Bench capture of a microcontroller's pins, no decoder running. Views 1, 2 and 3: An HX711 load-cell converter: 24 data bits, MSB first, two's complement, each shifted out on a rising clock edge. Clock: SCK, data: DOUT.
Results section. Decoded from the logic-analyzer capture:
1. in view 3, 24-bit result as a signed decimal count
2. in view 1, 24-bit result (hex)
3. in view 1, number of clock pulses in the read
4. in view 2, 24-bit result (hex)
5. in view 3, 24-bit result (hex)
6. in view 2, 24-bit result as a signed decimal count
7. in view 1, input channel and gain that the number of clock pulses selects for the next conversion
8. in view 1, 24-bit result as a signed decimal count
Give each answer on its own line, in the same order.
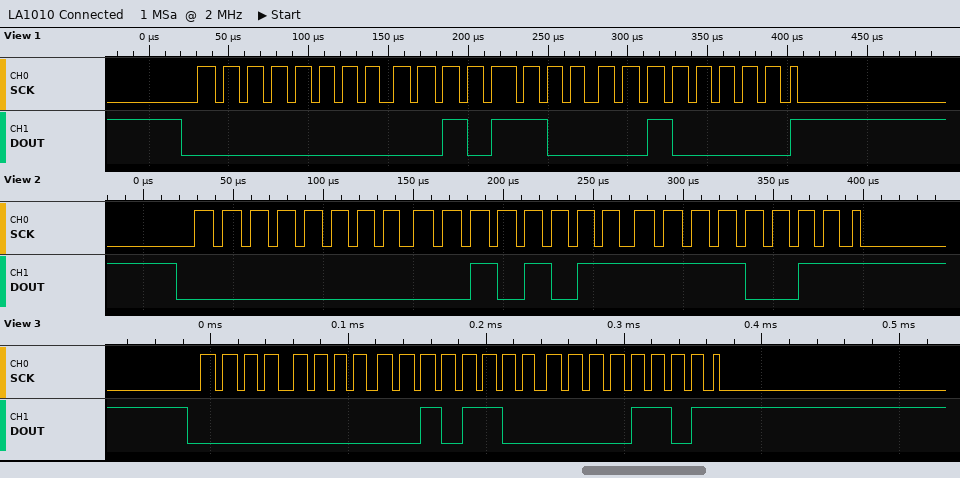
11277
0x002C20
25
0x002BF3
0x002C0D
11251
channel A, gain 128
11296
